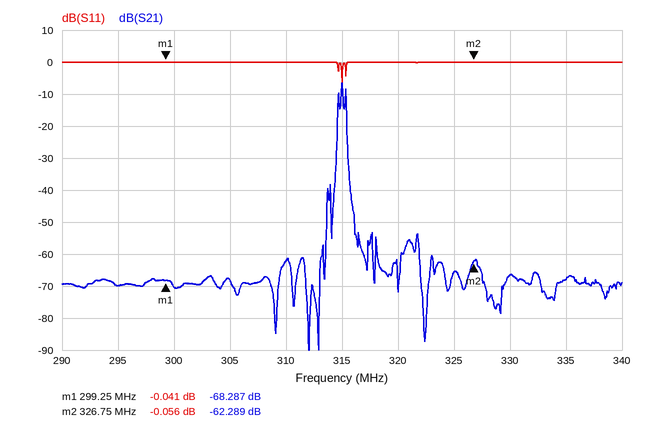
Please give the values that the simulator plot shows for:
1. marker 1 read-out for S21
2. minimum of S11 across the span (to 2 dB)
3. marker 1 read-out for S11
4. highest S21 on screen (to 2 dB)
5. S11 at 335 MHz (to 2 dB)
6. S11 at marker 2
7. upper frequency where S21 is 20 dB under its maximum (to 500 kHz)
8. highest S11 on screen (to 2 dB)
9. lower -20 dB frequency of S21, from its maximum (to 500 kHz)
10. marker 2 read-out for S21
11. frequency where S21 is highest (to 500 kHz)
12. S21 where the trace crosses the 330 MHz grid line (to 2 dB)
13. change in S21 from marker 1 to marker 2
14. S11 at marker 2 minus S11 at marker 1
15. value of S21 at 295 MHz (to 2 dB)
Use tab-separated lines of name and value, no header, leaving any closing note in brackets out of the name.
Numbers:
marker 1 read-out for S21	-68.287 dB
minimum of S11 across the span	-6 dB
marker 1 read-out for S11	-0.041 dB
highest S21 on screen	-6 dB
S11 at 335 MHz	0 dB
S11 at marker 2	-0.056 dB
upper frequency where S21 is 20 dB under its maximum	315.5 MHz
highest S11 on screen	0 dB
lower -20 dB frequency of S21, from its maximum	314.5 MHz
marker 2 read-out for S21	-62.289 dB
frequency where S21 is highest	315.0 MHz
S21 where the trace crosses the 330 MHz grid line	-66 dB
change in S21 from marker 1 to marker 2	5.998 dB
S11 at marker 2 minus S11 at marker 1	-0.015 dB
value of S21 at 295 MHz	-70 dB
